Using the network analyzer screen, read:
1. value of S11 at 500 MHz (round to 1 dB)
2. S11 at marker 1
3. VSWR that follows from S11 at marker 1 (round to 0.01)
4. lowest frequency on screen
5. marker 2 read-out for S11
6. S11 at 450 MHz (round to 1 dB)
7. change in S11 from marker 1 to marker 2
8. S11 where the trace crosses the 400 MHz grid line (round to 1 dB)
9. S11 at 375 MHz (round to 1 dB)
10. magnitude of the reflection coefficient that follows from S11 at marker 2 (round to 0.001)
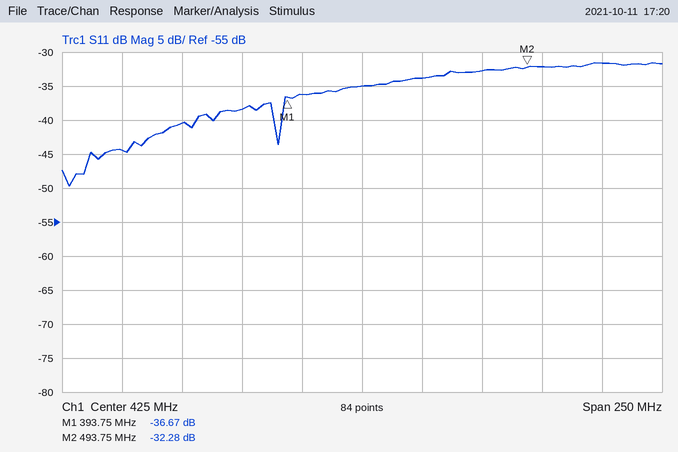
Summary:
-32 dB
-36.67 dB
1.03
300 MHz
-32.28 dB
-34 dB
4.39 dB
-36 dB
-38 dB
0.024
